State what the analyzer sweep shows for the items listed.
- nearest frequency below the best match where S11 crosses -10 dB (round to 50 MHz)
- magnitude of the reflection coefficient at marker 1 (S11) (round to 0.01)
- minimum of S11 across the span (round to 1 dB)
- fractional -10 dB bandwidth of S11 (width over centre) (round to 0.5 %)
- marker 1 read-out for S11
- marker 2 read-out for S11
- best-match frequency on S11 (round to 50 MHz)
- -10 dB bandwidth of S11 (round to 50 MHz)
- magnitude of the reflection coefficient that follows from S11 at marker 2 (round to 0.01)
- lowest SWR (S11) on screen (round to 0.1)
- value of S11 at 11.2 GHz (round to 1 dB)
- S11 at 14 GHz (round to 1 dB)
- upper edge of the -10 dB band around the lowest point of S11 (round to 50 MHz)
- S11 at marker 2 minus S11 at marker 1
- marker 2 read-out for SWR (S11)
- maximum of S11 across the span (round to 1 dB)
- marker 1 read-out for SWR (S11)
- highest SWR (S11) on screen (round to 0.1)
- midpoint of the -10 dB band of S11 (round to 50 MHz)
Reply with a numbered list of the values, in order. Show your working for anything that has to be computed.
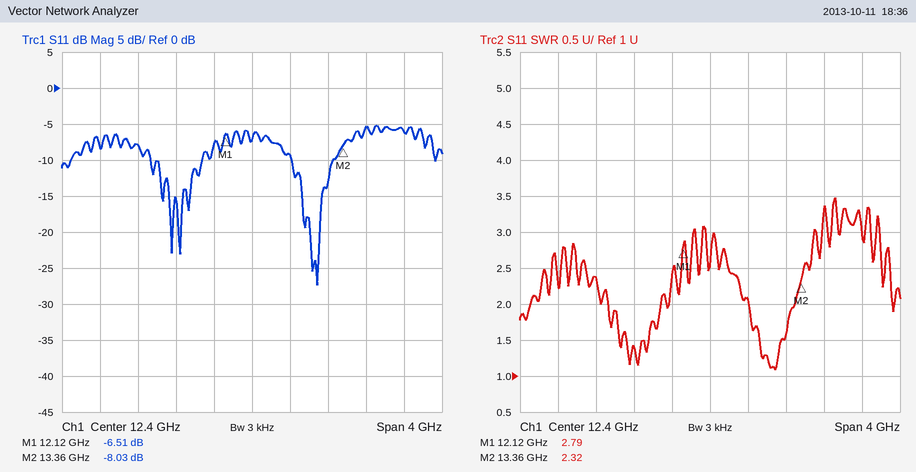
1. 12.80 GHz
2. 10^(-6.51/20) ≈ 0.47
3. -27 dB
4. 450 MHz / 13.025 GHz ≈ 3.5 %
5. -6.51 dB
6. -8.03 dB
7. 13.10 GHz
8. 13.25 GHz − 12.80 GHz = 450 MHz
9. 10^(-8.03/20) ≈ 0.40
10. 1.1
11. -8 dB
12. -6 dB
13. 13.25 GHz
14. -8.03 − (-6.51) = -1.52 dB
15. 2.32
16. -5 dB
17. 2.79
18. 3.5
19. 13.05 GHz
